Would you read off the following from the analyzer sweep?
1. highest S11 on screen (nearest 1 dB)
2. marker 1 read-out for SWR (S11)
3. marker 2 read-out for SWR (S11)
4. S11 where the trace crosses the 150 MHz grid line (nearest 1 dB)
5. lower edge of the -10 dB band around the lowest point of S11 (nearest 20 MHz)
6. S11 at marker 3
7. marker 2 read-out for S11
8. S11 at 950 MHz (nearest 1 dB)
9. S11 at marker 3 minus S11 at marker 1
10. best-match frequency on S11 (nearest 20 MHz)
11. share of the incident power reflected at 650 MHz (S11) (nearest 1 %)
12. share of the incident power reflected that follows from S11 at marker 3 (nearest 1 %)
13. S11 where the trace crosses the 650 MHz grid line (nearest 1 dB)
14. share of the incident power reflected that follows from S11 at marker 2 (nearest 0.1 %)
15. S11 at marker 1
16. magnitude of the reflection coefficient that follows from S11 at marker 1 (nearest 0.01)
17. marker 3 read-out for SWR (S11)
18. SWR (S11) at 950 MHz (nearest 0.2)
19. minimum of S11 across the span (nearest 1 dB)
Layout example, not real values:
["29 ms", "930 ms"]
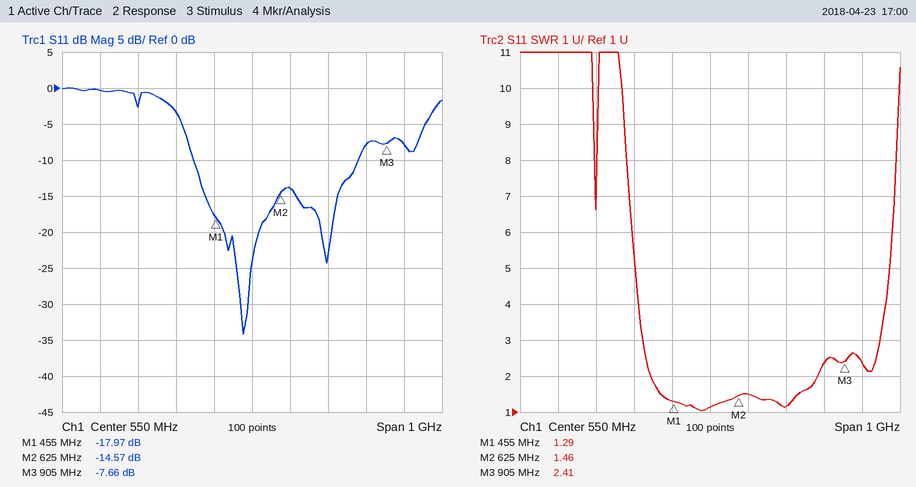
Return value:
["0 dB", "1.29", "1.46", "0 dB", "400 MHz", "-7.66 dB", "-14.57 dB", "-8 dB", "10.31 dB", "520 MHz", "4 %", "17 %", "-14 dB", "3.5 %", "-17.97 dB", "0.13", "2.41", "2.4", "-34 dB"]
